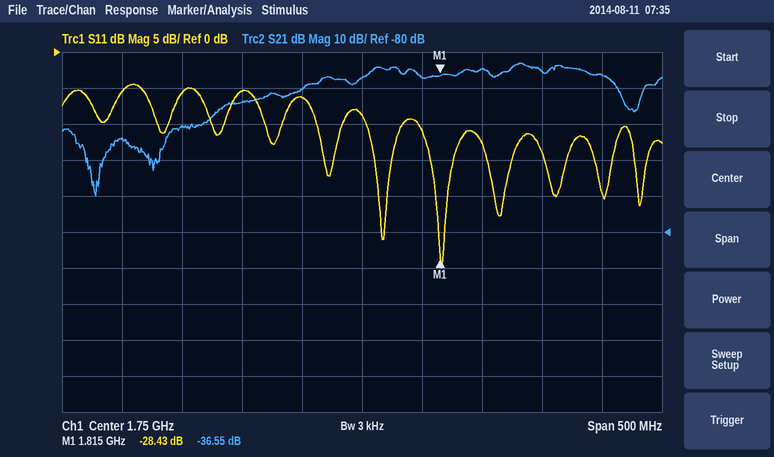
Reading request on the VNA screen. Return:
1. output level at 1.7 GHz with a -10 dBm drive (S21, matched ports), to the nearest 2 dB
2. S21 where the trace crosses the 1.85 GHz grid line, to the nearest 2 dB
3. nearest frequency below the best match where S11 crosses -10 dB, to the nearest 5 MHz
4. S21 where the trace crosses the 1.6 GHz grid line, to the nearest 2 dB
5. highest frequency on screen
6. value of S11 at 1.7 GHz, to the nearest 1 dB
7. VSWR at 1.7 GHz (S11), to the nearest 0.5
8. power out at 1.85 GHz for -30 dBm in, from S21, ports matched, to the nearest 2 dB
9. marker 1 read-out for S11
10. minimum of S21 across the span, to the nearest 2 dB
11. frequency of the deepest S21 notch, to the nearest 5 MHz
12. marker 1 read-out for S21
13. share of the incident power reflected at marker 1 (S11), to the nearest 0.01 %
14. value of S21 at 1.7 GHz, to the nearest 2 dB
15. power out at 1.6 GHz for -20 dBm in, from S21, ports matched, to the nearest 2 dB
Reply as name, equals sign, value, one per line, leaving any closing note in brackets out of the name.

output level at 1.7 GHz with a -10 dBm drive (S21, matched ports), to the nearest 2 dB = -50 dBm
S21 where the trace crosses the 1.85 GHz grid line, to the nearest 2 dB = -34 dB
nearest frequency below the best match where S11 crosses -10 dB, to the nearest 5 MHz = 1.795 GHz
S21 where the trace crosses the 1.6 GHz grid line, to the nearest 2 dB = -50 dB
highest frequency on screen = 2 GHz
value of S11 at 1.7 GHz, to the nearest 1 dB = -6 dB
VSWR at 1.7 GHz (S11), to the nearest 0.5 = 3.0
power out at 1.85 GHz for -30 dBm in, from S21, ports matched, to the nearest 2 dB = -64 dBm
marker 1 read-out for S11 = -28.43 dB
minimum of S21 across the span, to the nearest 2 dB = -70 dB
frequency of the deepest S21 notch, to the nearest 5 MHz = 1.530 GHz
marker 1 read-out for S21 = -36.55 dB
share of the incident power reflected at marker 1 (S11), to the nearest 0.01 % = 0.14 %
value of S21 at 1.7 GHz, to the nearest 2 dB = -40 dB
power out at 1.6 GHz for -20 dBm in, from S21, ports matched, to the nearest 2 dB = -70 dBm
